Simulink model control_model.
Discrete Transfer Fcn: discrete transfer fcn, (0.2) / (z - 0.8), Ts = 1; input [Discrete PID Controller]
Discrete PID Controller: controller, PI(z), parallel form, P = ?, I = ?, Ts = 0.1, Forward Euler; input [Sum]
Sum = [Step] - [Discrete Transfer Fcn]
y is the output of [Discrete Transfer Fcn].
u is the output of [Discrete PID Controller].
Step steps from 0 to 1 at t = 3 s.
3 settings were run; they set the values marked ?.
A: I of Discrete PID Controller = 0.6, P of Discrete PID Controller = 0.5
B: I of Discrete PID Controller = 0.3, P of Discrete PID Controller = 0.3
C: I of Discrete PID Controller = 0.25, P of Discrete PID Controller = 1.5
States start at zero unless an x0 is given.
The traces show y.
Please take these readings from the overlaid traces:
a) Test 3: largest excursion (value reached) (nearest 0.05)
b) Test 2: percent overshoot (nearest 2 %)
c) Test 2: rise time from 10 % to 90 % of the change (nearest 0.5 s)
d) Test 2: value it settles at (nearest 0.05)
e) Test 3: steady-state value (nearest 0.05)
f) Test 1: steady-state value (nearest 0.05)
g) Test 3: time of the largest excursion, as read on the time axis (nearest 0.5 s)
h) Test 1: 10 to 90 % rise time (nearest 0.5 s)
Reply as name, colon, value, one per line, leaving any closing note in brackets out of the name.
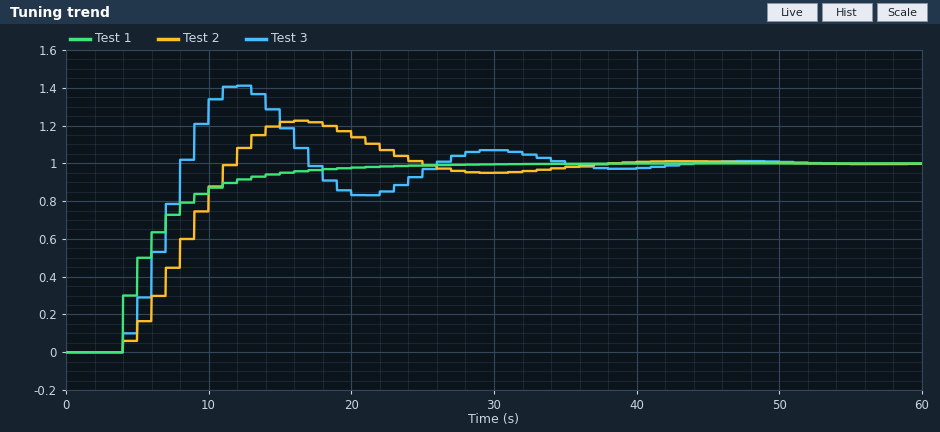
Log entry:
Test 3: largest excursion (value reached): 1.40
Test 2: percent overshoot: 22 %
Test 2: rise time from 10 % to 90 % of the change: 6.0 s
Test 2: value it settles at: 1.00
Test 3: steady-state value: 1.00
Test 1: steady-state value: 1.00
Test 3: time of the largest excursion, as read on the time axis: 12.0 s
Test 1: 10 to 90 % rise time: 8.0 s
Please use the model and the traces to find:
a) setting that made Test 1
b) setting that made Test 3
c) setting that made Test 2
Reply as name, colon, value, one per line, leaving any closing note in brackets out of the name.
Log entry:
setting that made Test 1: C
setting that made Test 3: A
setting that made Test 2: B
